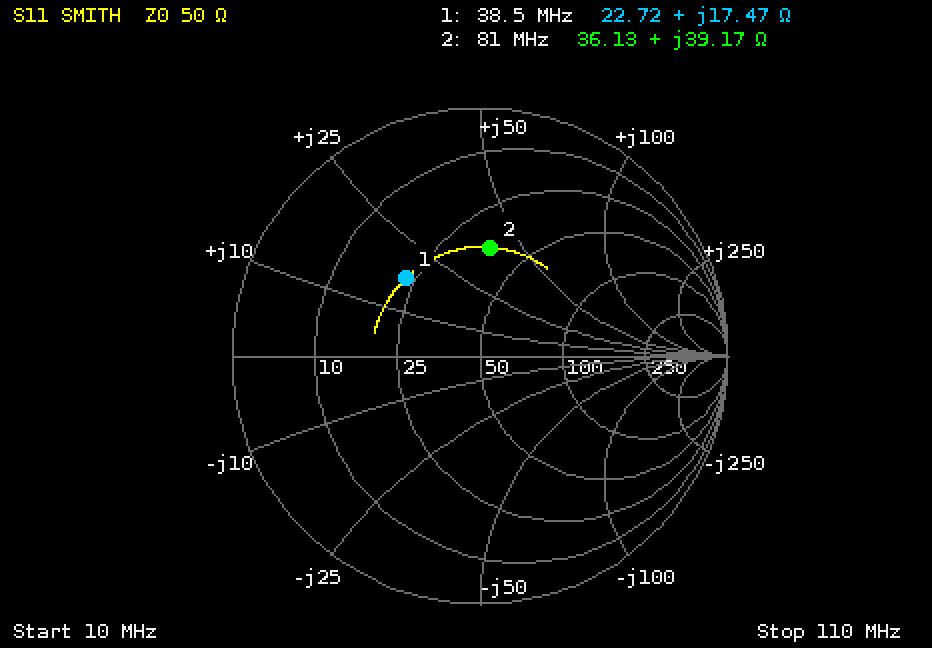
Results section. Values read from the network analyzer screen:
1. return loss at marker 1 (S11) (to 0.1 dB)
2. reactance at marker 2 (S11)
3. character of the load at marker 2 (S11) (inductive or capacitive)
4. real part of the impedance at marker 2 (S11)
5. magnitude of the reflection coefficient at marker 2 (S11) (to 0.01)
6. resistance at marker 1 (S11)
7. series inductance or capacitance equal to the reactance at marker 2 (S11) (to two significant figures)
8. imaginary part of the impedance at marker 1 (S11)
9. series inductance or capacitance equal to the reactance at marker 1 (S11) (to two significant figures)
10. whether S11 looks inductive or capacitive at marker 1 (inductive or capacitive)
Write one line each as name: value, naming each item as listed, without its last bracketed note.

return loss at marker 1 (S11): 7.3 dB
reactance at marker 2: +39.17 Ω
character of the load at marker 2 (S11): inductive
real part of the impedance at marker 2: 36.13 Ω
magnitude of the reflection coefficient at marker 2 (S11): 0.44
resistance at marker 1: 22.72 Ω
series inductance or capacitance equal to the reactance at marker 2 (S11): 77 nH
imaginary part of the impedance at marker 1: +17.47 Ω
series inductance or capacitance equal to the reactance at marker 1 (S11): 72 nH
whether S11 looks inductive or capacitive at marker 1: inductive
